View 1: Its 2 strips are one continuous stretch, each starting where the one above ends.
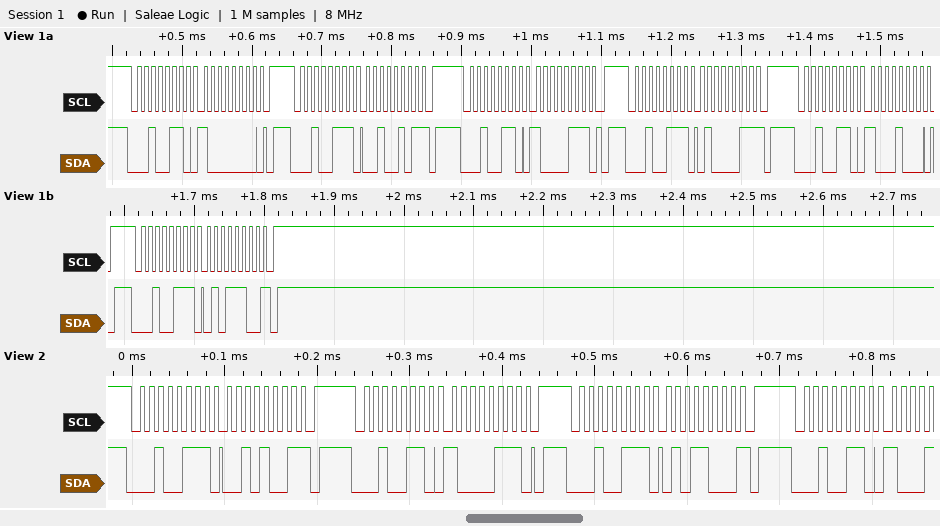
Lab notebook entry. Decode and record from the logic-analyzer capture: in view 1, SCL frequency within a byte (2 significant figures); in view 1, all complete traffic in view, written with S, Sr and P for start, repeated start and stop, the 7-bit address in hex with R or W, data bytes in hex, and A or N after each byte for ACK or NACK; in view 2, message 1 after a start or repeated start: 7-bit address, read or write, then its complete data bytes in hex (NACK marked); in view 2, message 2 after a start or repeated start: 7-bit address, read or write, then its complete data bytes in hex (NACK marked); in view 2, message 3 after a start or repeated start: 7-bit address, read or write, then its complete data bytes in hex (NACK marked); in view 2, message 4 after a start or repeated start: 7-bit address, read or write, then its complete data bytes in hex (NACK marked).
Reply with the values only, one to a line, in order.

100 kHz
S 13W A 80 A P S 13R A 25 N P S 13W A 87 A P S 13R A 43 N P S 13W A 88 A P S 13R A 5C N P
0x13 read: 29 NACK
0x13 write: 87
0x13 read: 58 NACK
0x13 write
